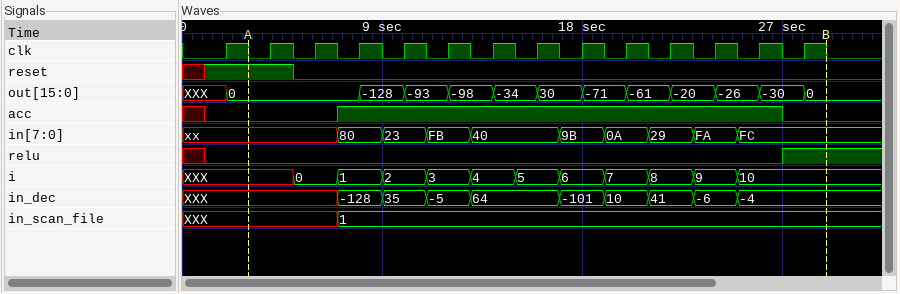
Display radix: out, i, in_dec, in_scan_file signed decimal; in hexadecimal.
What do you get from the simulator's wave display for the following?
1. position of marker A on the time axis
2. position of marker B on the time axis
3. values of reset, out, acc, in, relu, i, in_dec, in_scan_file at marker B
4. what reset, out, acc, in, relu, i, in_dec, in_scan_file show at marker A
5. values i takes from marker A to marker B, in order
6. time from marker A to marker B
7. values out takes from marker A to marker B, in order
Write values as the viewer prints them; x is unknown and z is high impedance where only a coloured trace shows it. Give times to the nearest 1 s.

3 s
29 s
reset=0, out=0, acc=0, in=FC, relu=1, i=10, in_dec=-4, in_scan_file=1
reset=1, out=0, acc=0, in=xx, relu=0, i=XXX, in_dec=XXX, in_scan_file=XXX
XXX, 0, 1, 2, 3, 4, 5, 6, 7, 8, 9, 10
26 s
0, -128, -93, -98, -34, 30, -71, -61, -20, -26, -30, 0
